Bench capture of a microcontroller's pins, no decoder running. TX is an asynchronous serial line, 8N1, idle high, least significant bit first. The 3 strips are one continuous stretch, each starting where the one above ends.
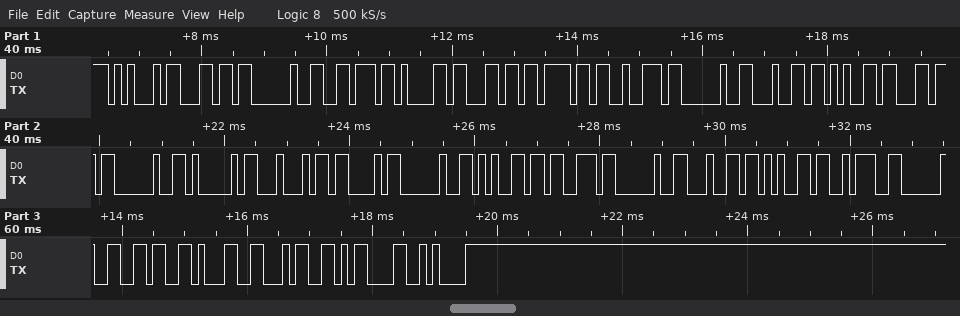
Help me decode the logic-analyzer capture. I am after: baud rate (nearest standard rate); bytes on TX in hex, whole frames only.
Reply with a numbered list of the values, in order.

1. 9600 baud
2. 45 6C 20 76 61 6C 6F 72 20 64 65 6C 20 41 44 43 20 65 73 20 64 65 3A 20 36 31 34 0D 0A
